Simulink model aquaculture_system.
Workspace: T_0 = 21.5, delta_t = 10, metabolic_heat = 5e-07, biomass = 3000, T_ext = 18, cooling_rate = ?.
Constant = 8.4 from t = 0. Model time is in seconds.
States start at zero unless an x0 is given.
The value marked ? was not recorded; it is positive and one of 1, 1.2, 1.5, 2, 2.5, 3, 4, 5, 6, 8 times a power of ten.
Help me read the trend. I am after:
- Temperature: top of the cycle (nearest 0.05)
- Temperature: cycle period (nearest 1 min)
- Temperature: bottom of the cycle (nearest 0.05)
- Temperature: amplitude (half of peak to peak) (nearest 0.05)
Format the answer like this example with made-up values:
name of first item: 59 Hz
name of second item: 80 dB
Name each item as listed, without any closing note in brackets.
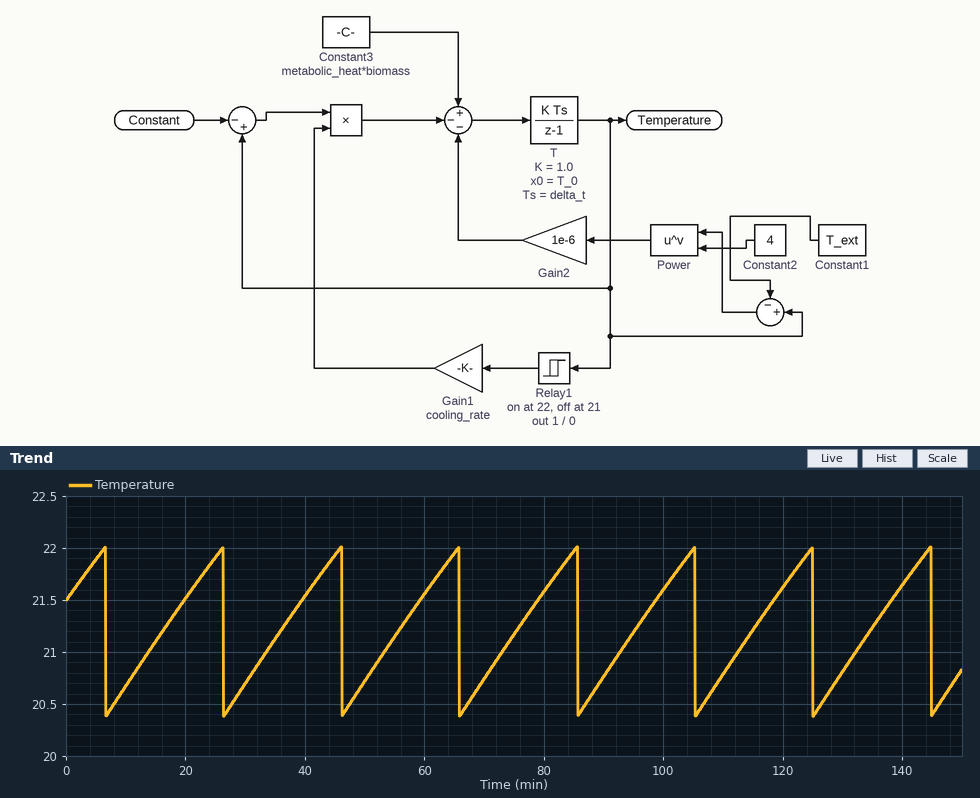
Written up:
Temperature: top of the cycle: 22.00
Temperature: cycle period: 20 min
Temperature: bottom of the cycle: 20.40
Temperature: amplitude (half of peak to peak): 0.80
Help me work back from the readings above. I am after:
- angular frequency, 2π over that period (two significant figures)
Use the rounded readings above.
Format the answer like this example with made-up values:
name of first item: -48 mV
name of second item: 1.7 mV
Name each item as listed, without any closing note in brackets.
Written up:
angular frequency, 2π over that period: 0.31 rad/min
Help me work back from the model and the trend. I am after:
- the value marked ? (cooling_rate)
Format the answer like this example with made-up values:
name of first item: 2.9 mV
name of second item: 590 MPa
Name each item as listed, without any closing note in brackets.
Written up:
the value marked ?: 0.012
